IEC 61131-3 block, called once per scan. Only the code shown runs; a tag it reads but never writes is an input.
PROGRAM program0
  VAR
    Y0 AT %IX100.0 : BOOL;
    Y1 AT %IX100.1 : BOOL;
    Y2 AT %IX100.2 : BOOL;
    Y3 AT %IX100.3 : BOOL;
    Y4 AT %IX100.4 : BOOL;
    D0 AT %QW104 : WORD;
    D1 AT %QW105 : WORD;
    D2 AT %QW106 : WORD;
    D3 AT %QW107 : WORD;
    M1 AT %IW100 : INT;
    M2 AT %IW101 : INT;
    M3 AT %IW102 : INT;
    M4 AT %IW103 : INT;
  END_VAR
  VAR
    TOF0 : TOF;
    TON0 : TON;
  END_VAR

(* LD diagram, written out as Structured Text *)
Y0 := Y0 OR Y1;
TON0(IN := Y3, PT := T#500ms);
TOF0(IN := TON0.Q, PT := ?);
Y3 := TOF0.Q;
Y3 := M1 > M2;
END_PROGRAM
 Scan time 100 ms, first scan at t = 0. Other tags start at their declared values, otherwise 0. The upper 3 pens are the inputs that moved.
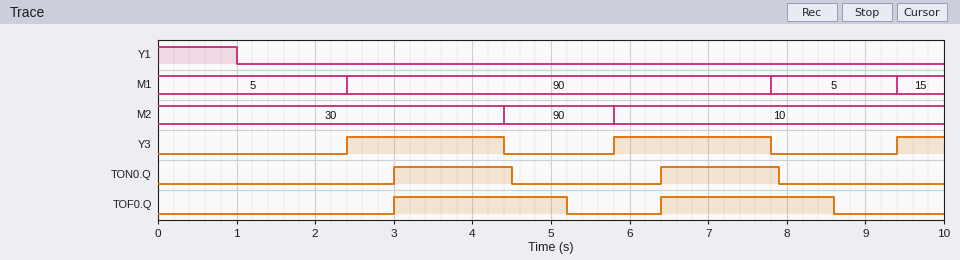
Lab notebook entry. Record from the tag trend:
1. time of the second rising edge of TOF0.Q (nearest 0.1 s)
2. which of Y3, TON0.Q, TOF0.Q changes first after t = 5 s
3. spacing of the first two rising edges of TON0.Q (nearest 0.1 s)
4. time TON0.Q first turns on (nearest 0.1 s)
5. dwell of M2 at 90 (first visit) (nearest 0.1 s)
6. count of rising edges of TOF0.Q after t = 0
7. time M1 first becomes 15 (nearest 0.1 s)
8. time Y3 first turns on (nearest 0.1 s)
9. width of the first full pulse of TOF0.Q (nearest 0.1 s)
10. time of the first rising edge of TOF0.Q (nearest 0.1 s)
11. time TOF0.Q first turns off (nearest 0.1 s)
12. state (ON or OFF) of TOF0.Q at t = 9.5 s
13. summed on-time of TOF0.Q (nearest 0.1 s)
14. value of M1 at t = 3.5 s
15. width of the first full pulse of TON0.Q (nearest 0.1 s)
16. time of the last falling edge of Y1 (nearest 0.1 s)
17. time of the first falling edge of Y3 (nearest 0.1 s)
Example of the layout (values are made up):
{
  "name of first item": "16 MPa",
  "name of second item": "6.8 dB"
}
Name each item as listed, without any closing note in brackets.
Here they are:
{
  "time of the second rising edge of TOF0.Q": "6.4 s",
  "which of Y3, TON0.Q, TOF0.Q changes first after t = 5 s": "TOF0.Q",
  "spacing of the first two rising edges of TON0.Q": "3.4 s",
  "time TON0.Q first turns on": "3.0 s",
  "dwell of M2 at 90 (first visit)": "1.4 s",
  "count of rising edges of TOF0.Q after t = 0": "2",
  "time M1 first becomes 15": "9.4 s",
  "time Y3 first turns on": "2.4 s",
  "width of the first full pulse of TOF0.Q": "2.2 s",
  "time of the first rising edge of TOF0.Q": "3.0 s",
  "time TOF0.Q first turns off": "5.2 s",
  "state (ON or OFF) of TOF0.Q at t = 9.5 s": "OFF",
  "summed on-time of TOF0.Q": "4.4 s",
  "value of M1 at t = 3.5 s": "90",
  "width of the first full pulse of TON0.Q": "1.5 s",
  "time of the last falling edge of Y1": "1.0 s",
  "time of the first falling edge of Y3": "4.4 s"
}
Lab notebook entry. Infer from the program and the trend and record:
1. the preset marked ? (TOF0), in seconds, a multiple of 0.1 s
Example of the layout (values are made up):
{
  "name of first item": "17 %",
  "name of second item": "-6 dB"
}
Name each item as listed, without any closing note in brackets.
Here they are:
{
  "the preset marked ? (TOF0), in seconds, a multiple of 0.1 s": "0.7 s"
}
